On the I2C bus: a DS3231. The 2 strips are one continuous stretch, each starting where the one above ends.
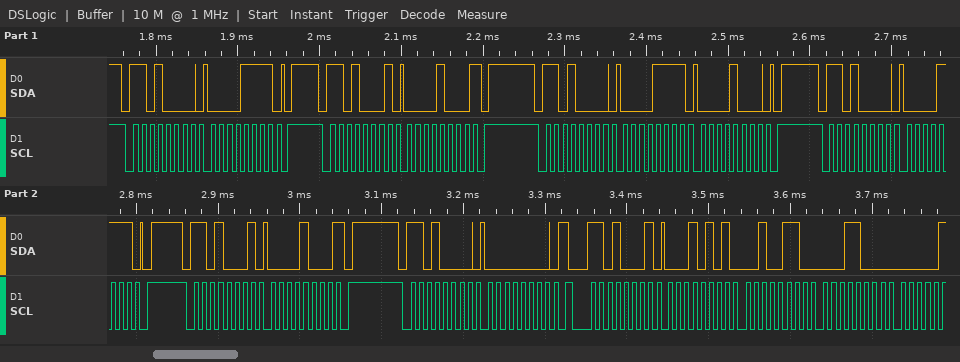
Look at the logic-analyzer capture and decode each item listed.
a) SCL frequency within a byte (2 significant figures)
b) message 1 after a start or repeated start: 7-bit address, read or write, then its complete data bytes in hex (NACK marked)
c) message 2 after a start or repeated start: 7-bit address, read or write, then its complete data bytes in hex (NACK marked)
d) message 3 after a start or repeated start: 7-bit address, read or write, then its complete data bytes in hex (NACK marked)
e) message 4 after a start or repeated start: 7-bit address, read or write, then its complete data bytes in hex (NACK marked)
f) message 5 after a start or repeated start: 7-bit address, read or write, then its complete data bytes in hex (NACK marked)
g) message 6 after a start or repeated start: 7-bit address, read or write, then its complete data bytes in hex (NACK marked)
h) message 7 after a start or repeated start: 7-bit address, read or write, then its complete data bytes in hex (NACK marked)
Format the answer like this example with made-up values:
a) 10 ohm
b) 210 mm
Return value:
a) 100 kHz
b) 0x68 write: 0F
c) 0x68 read: 08 NACK
d) 0x68 write: 0F 08
e) 0x68 write: 0F
f) 0x68 read: 08 NACK
g) 0x68 write: 00
h) 0x68 read: 15 26 18
